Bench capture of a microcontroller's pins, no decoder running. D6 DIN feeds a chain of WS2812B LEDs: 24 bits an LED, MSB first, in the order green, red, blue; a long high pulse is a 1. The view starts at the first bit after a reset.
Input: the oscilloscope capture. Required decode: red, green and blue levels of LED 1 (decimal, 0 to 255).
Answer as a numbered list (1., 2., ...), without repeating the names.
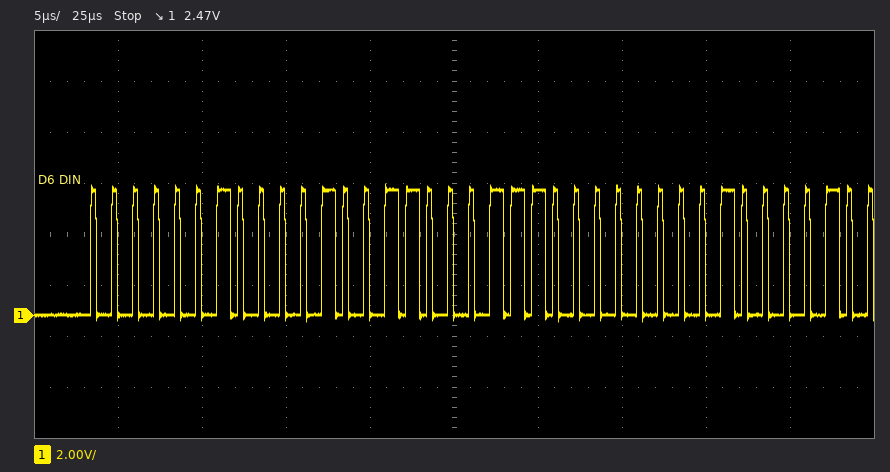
1. 19, 2, 28
